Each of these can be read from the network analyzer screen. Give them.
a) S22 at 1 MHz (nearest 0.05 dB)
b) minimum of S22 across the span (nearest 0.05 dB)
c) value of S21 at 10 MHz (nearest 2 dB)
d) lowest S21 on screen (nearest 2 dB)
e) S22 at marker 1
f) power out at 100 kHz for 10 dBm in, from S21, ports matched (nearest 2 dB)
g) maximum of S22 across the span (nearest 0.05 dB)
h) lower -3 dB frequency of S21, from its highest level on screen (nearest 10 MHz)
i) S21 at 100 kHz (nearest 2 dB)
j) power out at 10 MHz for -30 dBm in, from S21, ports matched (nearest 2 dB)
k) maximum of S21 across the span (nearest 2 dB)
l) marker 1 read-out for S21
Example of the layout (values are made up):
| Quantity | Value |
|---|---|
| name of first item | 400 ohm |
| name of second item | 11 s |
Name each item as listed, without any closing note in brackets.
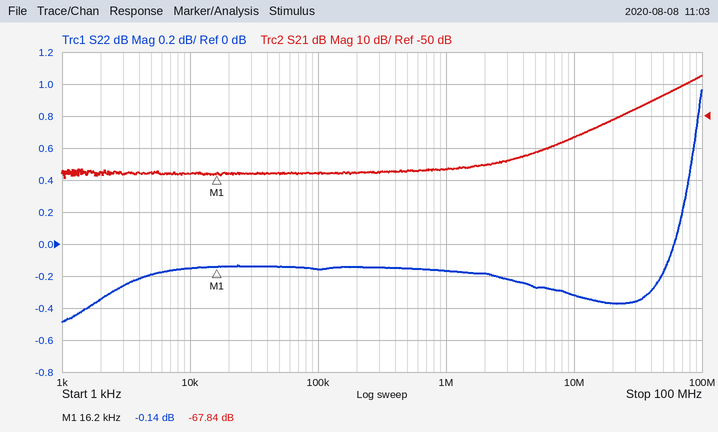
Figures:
| Quantity | Value |
|---|---|
| S22 at 1 MHz | -0.15 dB |
| minimum of S22 across the span | -0.50 dB |
| value of S21 at 10 MHz | -56 dB |
| lowest S21 on screen | -70 dB |
| S22 at marker 1 | -0.14 dB |
| power out at 100 kHz for 10 dBm in, from S21, ports matched | -58 dBm |
| maximum of S22 across the span | 0.95 dB |
| lower -3 dB frequency of S21, from its highest level on screen | 70 MHz |
| S21 at 100 kHz | -68 dB |
| power out at 10 MHz for -30 dBm in, from S21, ports matched | -86 dBm |
| maximum of S21 across the span | -38 dB |
| marker 1 read-out for S21 | -67.84 dB |
